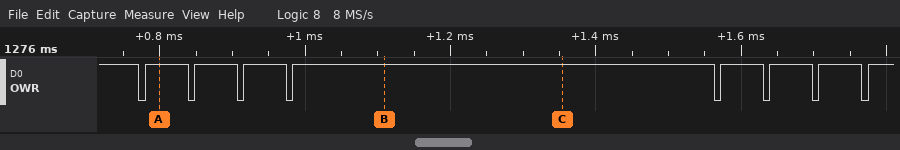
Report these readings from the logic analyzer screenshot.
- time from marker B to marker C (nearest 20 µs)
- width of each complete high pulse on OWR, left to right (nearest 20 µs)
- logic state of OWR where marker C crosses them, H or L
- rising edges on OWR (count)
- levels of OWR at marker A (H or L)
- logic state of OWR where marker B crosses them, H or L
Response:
240 µs
60 µs, 60 µs, 60 µs, 580 µs, 60 µs, 60 µs, 60 µs
OWR=H
8
OWR=H
OWR=H
